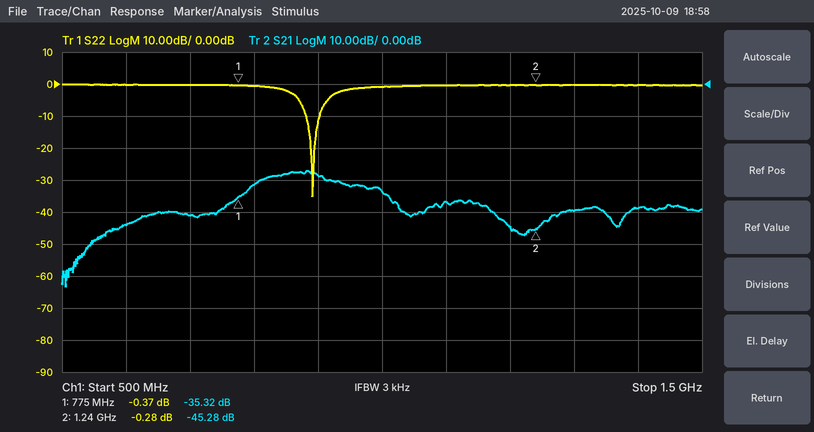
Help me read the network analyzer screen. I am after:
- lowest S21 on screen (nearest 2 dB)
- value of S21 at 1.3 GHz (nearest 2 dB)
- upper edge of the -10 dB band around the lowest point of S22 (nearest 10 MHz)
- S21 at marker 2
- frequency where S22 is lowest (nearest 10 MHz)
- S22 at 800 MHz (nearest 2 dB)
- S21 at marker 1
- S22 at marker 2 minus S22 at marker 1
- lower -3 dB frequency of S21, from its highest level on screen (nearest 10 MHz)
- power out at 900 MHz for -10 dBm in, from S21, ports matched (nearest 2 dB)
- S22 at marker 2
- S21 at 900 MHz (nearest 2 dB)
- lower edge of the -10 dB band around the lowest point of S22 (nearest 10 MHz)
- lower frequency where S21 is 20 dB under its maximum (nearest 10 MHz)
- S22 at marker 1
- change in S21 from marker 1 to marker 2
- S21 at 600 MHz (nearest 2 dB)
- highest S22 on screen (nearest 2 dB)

-64 dB
-40 dB
900 MHz
-45.28 dB
890 MHz
0 dB
-35.32 dB
0.09 dB
810 MHz
-38 dBm
-0.28 dB
-28 dB
880 MHz
570 MHz
-0.37 dB
-9.96 dB
-44 dB
0 dB
